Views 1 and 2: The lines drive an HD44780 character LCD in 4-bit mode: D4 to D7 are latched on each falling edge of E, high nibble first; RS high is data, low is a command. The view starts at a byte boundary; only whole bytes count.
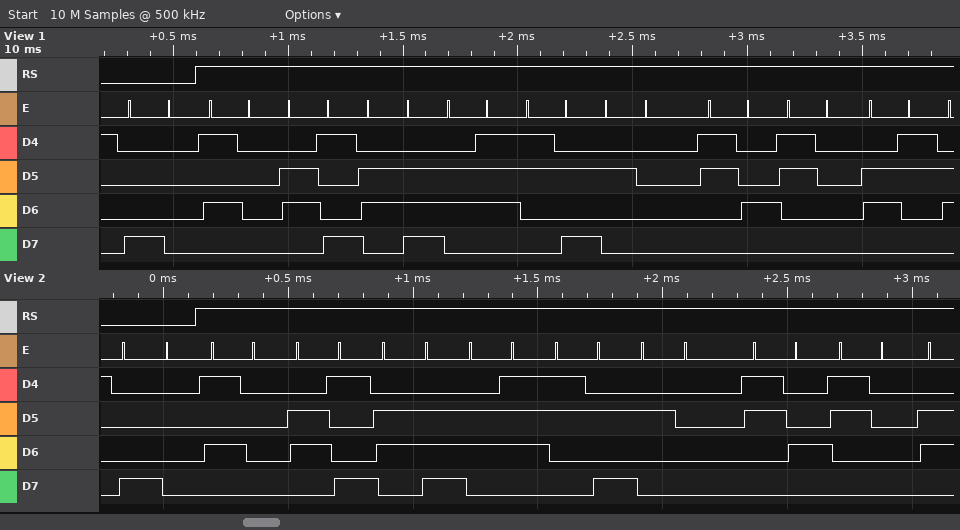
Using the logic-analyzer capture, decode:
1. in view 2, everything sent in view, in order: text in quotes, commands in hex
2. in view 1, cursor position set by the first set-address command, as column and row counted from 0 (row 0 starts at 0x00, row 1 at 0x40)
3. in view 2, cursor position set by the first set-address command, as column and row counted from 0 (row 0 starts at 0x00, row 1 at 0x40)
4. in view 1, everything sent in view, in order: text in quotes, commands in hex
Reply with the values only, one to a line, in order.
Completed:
0x80 "Ping: 40"
column 0, row 0
column 0, row 0
0x80 "Ping: 40c"
